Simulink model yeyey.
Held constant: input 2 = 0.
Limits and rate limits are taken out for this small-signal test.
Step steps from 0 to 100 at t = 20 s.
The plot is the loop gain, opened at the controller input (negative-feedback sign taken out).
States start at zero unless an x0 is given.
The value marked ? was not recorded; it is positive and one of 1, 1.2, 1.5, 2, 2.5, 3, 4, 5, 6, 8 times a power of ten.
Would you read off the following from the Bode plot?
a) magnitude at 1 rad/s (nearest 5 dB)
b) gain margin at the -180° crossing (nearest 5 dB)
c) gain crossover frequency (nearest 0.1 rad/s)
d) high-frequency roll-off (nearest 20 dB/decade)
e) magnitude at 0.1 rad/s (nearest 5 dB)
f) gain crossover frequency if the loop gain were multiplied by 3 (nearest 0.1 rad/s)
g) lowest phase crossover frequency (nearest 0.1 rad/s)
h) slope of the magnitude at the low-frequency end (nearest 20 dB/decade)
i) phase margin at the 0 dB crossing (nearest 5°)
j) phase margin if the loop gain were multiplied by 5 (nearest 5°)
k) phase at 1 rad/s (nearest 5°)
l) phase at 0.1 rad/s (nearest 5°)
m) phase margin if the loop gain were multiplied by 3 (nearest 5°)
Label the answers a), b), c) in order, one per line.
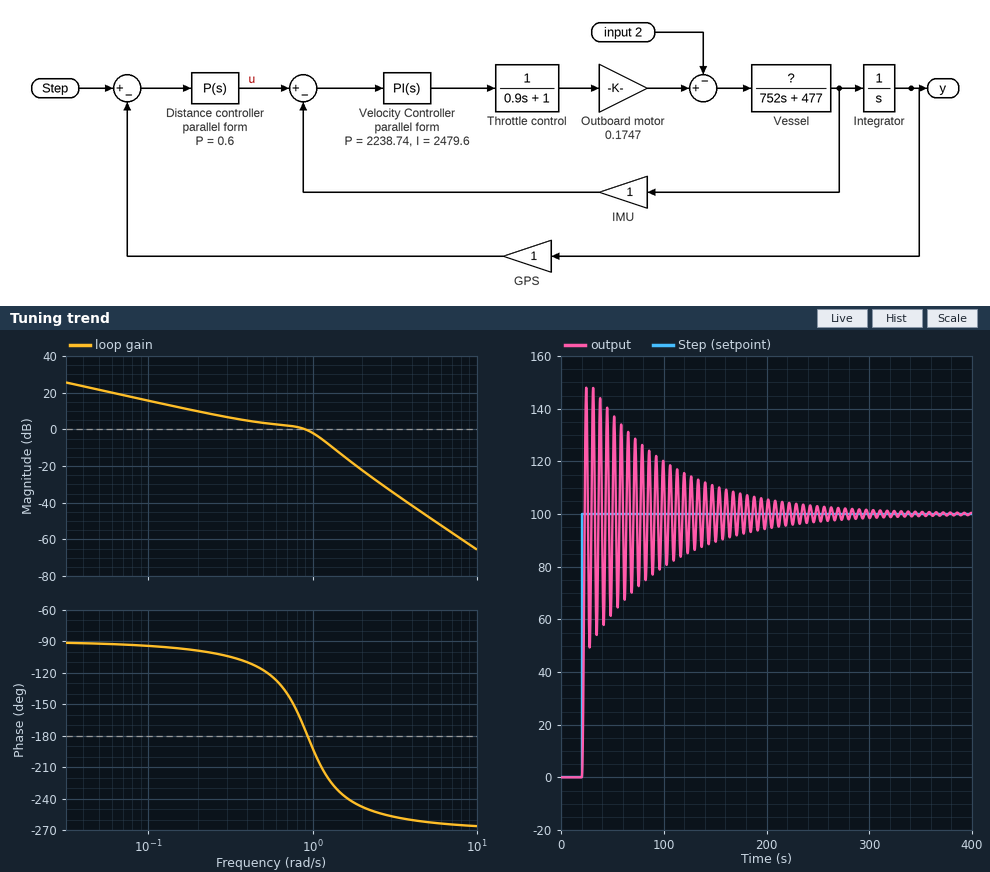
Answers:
a) 0 dB
b) 0 dB
c) 0.9 rad/s
d) -60 dB/decade
e) 15 dB
f) 1.3 rad/s
g) 0.9 rad/s
h) -20 dB/decade
i) 5°
j) -55°
k) -190°
l) -95°
m) -45°
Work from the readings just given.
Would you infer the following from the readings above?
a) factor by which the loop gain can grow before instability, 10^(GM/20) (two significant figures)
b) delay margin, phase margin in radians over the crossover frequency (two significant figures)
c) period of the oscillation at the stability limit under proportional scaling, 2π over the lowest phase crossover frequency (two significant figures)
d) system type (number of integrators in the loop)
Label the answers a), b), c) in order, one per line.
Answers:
a) 1.0
b) 0.097 s
c) 7.0 s
d) 1
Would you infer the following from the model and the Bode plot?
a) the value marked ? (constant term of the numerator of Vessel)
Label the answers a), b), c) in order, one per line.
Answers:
a) 1.5
